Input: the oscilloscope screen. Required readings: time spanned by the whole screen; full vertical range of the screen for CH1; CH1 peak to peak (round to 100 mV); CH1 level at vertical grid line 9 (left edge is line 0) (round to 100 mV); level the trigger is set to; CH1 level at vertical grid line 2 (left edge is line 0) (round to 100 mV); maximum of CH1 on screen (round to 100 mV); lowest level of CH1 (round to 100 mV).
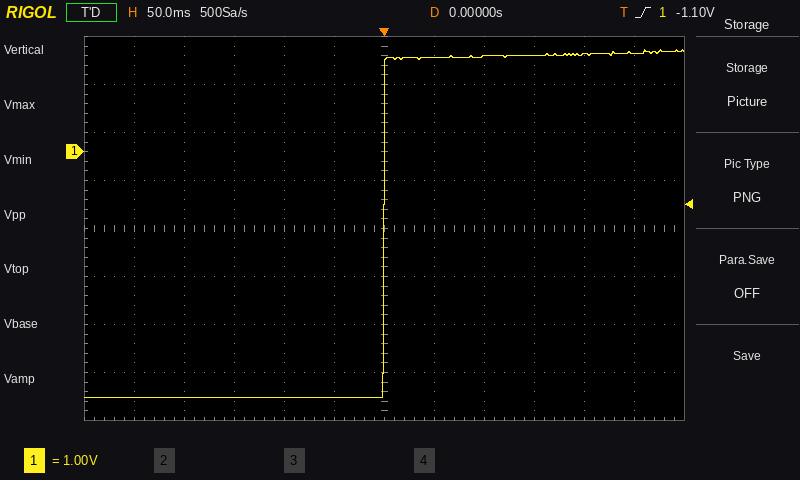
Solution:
600 ms
8 V
7.2 V
2.0 V
-1.10 V
-5.1 V
2.1 V
-5.1 V
